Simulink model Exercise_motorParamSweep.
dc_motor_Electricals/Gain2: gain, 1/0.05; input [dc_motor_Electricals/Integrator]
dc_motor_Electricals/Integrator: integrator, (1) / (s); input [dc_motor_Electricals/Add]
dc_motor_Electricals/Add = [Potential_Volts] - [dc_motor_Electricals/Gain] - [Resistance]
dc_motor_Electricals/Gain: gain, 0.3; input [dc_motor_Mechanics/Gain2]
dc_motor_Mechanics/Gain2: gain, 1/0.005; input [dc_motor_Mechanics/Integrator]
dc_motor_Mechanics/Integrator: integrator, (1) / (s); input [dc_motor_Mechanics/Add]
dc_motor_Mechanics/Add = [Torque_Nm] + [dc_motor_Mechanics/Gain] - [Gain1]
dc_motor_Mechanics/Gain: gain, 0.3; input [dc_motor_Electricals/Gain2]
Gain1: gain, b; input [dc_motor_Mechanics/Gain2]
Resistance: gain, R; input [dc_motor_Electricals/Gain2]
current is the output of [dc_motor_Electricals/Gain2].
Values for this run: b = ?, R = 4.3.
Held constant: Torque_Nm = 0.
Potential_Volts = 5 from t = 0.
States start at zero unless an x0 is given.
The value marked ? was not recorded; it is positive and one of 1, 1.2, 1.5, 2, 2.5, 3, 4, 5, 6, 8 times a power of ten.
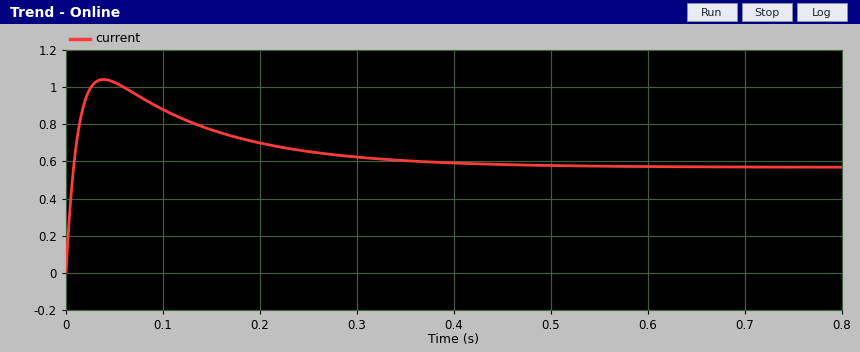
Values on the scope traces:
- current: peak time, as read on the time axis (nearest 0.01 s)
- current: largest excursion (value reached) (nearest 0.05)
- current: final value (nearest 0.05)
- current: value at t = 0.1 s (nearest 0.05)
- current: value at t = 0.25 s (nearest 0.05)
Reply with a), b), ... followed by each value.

a) 0.04 s
b) 1.05
c) 0.55
d) 0.90
e) 0.65
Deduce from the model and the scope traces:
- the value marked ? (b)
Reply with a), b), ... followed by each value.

a) 0.02
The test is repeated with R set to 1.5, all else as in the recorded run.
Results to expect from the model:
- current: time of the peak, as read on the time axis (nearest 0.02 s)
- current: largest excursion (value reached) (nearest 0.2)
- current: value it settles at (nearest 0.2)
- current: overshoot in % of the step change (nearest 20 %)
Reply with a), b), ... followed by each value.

a) 0.06 s
b) 2.2
c) 0.8
d) 180 %
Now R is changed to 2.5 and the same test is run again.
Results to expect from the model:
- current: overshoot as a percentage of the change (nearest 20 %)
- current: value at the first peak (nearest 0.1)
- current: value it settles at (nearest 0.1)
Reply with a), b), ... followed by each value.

a) 120 %
b) 1.6
c) 0.7
